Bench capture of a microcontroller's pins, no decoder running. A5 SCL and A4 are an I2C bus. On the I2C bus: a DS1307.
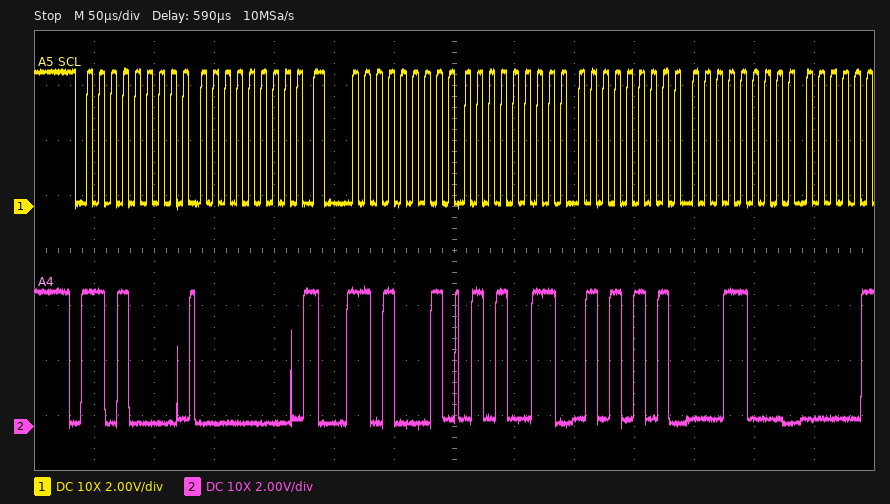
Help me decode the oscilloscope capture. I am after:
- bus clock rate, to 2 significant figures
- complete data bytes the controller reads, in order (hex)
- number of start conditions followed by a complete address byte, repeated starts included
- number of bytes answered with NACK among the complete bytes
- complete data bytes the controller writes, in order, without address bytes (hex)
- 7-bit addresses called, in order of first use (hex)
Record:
100 kHz
53 55 18
2
0
00
0x68
